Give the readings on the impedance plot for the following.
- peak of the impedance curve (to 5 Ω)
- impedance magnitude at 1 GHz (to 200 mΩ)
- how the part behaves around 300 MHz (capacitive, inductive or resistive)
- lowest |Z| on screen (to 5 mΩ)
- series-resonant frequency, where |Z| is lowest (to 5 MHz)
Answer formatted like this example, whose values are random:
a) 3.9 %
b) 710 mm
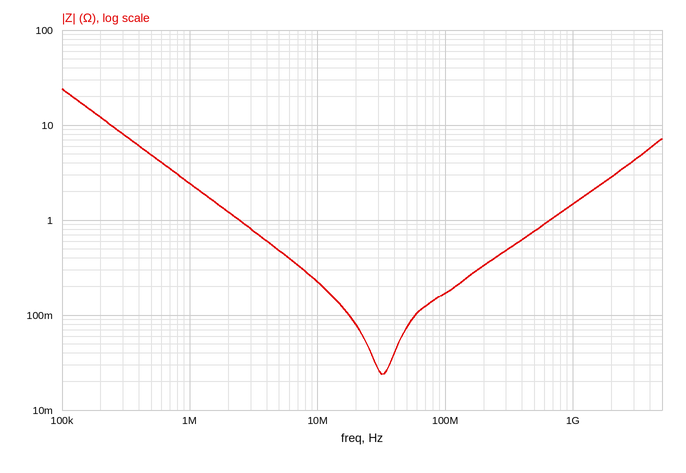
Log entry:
a) 25 Ω
b) 1.4 Ω
c) inductive
d) 25 mΩ
e) 30 MHz
